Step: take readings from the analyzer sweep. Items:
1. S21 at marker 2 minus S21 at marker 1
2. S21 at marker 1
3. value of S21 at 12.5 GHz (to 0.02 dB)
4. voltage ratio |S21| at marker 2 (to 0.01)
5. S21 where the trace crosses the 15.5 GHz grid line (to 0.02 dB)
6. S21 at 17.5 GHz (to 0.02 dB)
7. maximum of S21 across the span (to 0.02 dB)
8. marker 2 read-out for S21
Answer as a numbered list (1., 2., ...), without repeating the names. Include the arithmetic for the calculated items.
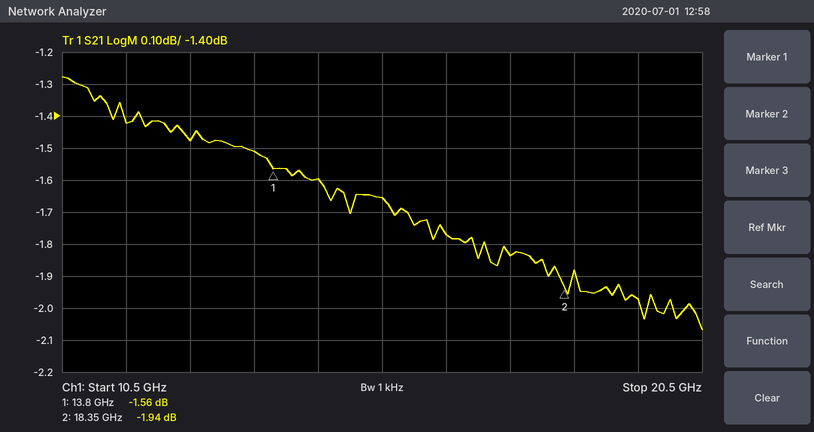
1. -1.94 − (-1.56) = -0.38 dB
2. -1.56 dB
3. -1.48 dB
4. 10^(-1.94/20) ≈ 0.80
5. -1.66 dB
6. -1.84 dB
7. -1.28 dB
8. -1.94 dB
